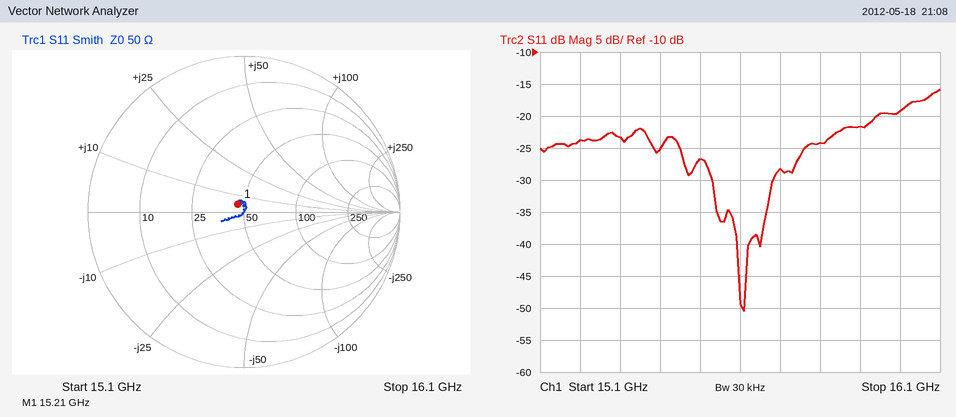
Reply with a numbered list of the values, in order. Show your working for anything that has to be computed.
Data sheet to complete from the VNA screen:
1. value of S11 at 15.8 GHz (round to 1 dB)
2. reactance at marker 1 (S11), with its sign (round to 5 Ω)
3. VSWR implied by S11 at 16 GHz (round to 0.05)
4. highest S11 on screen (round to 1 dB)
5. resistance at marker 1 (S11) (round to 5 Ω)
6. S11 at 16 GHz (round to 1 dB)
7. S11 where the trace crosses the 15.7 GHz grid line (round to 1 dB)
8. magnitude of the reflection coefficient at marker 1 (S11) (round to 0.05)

1. -24 dB
2. +5 Ω
3. |Γ| = 10^(-19/20) = 0.1122; VSWR = (1 + 0.1122)/(1 − 0.1122) ≈ 1.25
4. -16 dB
5. 45 Ω
6. -19 dB
7. -28 dB
8. 0.05
